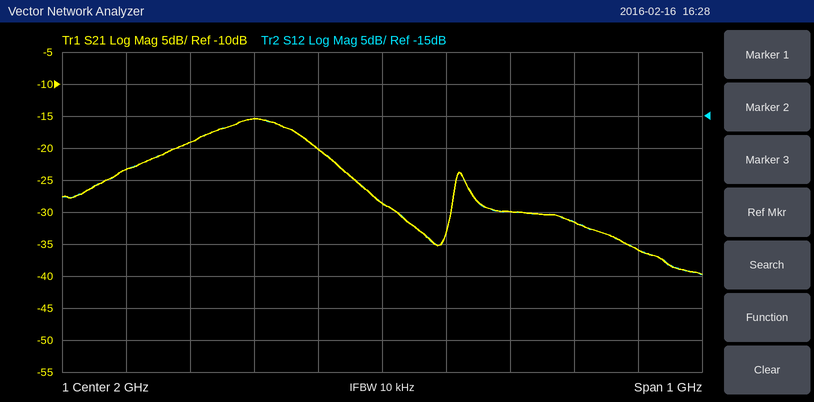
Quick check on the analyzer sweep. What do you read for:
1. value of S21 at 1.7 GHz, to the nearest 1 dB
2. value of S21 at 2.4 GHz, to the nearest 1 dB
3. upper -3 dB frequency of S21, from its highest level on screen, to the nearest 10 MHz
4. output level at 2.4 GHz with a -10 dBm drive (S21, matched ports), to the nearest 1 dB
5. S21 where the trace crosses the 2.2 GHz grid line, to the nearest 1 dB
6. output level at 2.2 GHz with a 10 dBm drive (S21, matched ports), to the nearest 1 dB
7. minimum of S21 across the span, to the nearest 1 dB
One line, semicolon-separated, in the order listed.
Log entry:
-19 dB; -36 dB; 1.88 GHz; -46 dBm; -30 dB; -20 dBm; -40 dB
